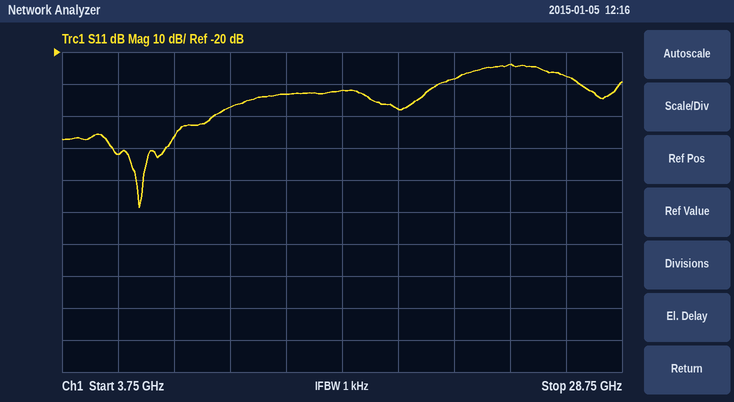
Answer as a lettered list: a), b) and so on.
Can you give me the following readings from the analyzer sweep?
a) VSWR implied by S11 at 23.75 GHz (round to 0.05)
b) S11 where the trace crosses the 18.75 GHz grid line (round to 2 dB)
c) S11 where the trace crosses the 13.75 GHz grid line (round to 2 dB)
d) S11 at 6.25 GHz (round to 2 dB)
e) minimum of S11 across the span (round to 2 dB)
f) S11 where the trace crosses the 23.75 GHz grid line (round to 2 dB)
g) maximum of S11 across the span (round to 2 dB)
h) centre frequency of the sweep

a) 1.15
b) -38 dB
c) -34 dB
d) -52 dB
e) -68 dB
f) -24 dB
g) -24 dB
h) 16.25 GHz
